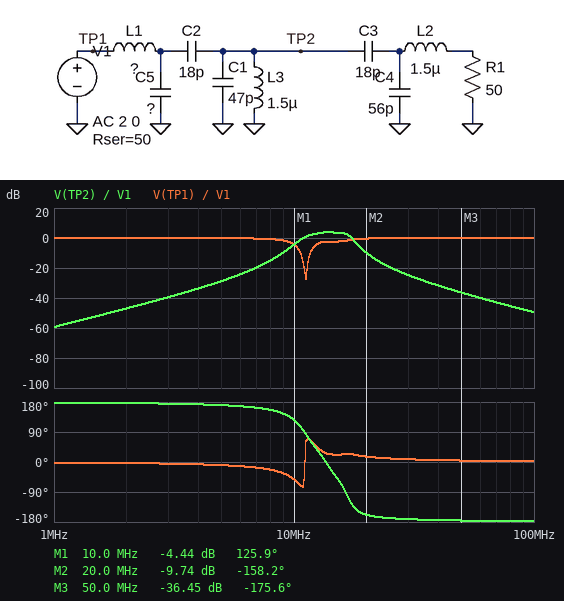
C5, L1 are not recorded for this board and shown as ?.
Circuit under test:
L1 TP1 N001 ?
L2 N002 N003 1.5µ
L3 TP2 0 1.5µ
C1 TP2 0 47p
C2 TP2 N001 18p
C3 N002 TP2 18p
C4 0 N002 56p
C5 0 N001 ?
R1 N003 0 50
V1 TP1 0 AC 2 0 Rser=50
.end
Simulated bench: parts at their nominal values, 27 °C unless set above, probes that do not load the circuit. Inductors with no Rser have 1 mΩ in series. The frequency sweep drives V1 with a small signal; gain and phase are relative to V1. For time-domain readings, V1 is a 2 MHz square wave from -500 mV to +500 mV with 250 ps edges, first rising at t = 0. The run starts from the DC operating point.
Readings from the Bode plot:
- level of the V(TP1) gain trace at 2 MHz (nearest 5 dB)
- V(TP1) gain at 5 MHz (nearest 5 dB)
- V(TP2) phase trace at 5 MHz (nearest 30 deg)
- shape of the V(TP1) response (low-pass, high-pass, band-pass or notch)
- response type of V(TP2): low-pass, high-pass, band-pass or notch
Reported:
0 dB
0 dB
180 deg
notch
band-pass
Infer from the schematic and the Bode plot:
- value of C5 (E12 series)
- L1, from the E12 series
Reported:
68 pF
2.2 µH
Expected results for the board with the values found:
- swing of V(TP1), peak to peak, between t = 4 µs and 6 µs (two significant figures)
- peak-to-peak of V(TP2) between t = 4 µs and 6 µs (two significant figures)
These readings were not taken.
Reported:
1.3 V
530 mV
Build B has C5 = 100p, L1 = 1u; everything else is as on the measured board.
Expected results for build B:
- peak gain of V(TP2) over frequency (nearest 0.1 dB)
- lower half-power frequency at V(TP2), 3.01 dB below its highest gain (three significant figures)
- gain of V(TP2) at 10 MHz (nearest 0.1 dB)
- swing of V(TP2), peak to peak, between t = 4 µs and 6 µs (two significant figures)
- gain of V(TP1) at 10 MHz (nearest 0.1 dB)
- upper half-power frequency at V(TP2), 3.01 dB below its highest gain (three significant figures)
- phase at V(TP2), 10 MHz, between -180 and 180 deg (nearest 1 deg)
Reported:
6.1 dB
12.6 MHz
-9.5 dB
600 mV
-1.9 dB
17.5 MHz
142 deg
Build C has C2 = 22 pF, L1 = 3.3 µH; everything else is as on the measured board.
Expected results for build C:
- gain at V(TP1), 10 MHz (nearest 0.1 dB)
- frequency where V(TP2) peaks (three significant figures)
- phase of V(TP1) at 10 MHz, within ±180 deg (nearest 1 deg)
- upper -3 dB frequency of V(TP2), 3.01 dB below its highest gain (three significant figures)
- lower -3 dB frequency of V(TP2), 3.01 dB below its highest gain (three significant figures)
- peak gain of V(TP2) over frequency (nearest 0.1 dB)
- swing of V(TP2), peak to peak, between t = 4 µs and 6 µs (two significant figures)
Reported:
-3.9 dB
14.0 MHz
50 deg
16.5 MHz
12.4 MHz
0.8 dB
480 mV
